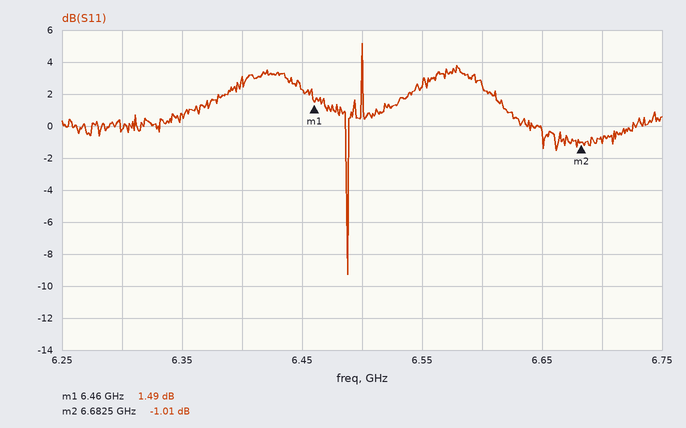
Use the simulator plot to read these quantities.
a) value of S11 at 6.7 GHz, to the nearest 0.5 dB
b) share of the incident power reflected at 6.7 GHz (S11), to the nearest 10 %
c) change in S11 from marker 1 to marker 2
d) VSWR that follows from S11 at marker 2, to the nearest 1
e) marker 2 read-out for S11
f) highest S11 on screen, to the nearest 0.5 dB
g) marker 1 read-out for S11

-1.0 dB
80 %
-2.50 dB
17
-1.01 dB
5.0 dB
1.49 dB
